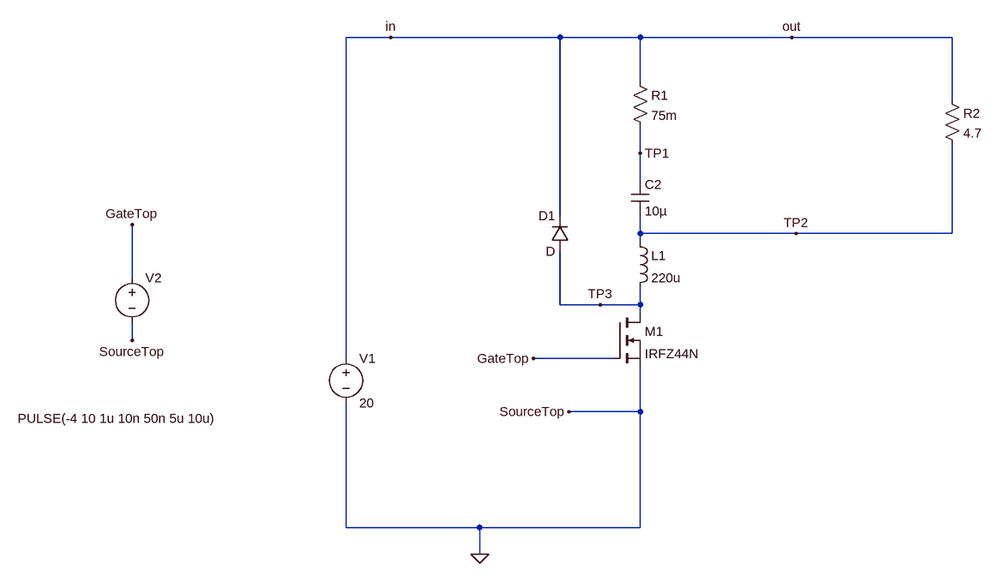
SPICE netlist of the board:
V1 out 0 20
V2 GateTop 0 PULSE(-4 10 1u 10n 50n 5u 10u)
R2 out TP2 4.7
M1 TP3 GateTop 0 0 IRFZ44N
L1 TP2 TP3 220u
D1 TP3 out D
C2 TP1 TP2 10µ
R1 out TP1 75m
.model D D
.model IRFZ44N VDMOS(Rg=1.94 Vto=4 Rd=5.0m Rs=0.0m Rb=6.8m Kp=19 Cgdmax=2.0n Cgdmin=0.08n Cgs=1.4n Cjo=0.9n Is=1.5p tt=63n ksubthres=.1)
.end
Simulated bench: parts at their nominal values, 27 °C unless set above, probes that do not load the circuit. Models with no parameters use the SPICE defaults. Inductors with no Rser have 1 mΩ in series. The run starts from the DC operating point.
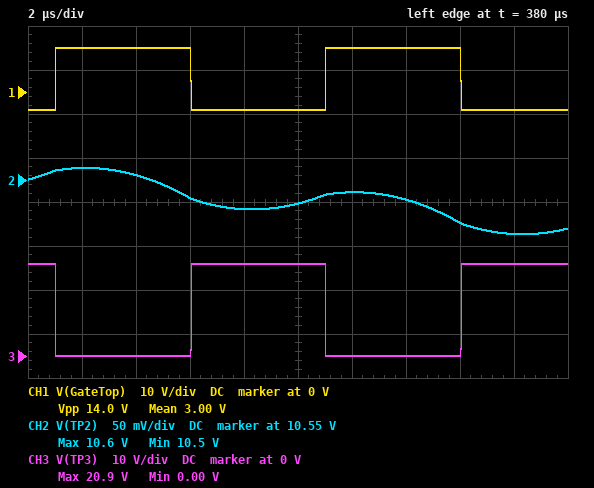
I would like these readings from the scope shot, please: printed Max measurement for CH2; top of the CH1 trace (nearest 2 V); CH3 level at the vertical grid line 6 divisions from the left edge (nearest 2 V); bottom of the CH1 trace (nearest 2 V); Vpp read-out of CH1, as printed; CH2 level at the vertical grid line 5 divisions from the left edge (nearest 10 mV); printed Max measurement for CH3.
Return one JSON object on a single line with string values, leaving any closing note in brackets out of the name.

{"printed Max measurement for CH2": "10.6 V", "top of the CH1 trace": "10 V", "CH3 level at the vertical grid line 6 divisions from the left edge": "0 V", "bottom of the CH1 trace": "-4 V", "Vpp read-out of CH1, as printed": "14.0 V", "CH2 level at the vertical grid line 5 divisions from the left edge": "10.52 V", "printed Max measurement for CH3": "20.9 V"}
